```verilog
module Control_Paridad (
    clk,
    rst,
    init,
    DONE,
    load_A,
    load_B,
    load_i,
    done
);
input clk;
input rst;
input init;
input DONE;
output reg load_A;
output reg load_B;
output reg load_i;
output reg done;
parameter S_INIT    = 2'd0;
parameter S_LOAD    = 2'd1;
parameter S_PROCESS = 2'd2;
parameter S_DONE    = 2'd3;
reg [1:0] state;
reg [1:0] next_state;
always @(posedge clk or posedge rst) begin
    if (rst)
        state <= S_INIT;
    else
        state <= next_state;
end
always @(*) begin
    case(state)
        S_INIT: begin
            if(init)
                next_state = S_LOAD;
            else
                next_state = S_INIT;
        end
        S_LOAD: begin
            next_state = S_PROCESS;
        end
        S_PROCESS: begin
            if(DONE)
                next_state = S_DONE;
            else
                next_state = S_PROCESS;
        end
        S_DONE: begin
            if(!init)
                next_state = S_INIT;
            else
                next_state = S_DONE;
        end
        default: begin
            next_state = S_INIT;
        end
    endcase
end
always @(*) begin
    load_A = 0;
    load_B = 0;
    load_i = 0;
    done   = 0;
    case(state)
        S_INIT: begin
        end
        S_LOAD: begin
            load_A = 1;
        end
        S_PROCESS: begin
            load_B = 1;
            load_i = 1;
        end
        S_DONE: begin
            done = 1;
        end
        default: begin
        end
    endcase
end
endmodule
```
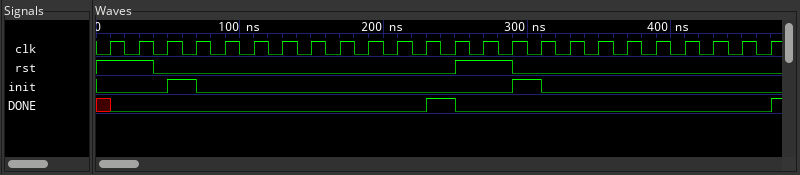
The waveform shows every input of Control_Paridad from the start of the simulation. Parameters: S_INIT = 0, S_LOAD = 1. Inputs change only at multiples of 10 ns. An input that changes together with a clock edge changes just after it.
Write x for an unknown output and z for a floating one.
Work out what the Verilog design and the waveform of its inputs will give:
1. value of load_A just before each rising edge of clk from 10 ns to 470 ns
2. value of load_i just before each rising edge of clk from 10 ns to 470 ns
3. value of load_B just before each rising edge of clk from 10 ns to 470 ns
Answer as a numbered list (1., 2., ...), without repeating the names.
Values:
1. 0 0 0 0 1 0 0 0 0 0 0 0 0 0 0 0 1 0 0 0 0 0 0 0
2. 0 0 0 0 0 1 1 1 1 1 1 1 1 0 0 0 0 1 1 1 1 1 1 1
3. 0 0 0 0 0 1 1 1 1 1 1 1 1 0 0 0 0 1 1 1 1 1 1 1
